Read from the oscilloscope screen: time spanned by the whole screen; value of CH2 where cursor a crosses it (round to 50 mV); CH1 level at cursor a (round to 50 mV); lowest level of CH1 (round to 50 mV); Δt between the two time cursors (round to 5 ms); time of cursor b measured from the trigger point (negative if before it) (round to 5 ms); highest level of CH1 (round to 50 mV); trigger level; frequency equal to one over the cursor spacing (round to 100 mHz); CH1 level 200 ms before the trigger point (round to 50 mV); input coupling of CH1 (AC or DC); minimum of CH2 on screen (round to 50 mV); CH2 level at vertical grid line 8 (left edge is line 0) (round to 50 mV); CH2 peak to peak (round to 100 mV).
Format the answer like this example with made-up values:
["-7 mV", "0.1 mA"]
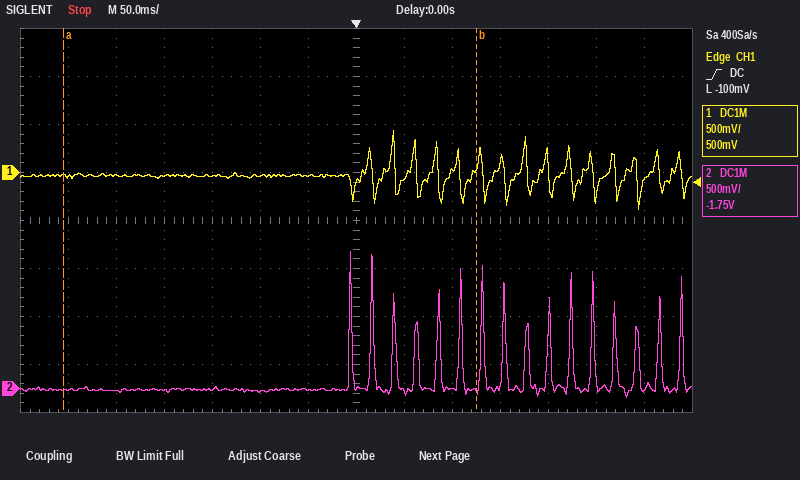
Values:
["700 ms", "0 mV", "-50 mV", "-400 mV", "430 ms", "+125 ms", "450 mV", "-100 mV", "2.3 Hz", "-50 mV", "DC", "-100 mV", "-50 mV", "1.50 V"]
